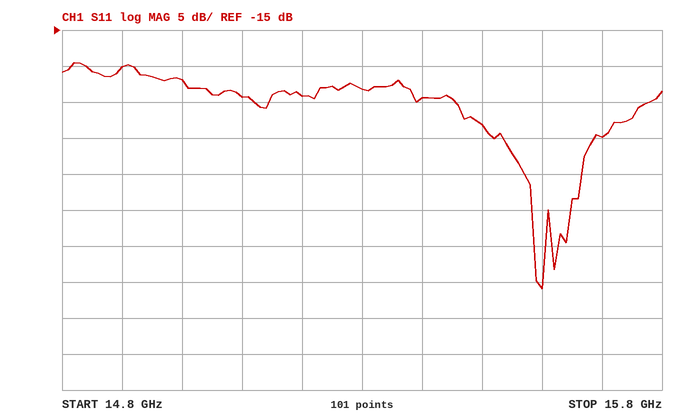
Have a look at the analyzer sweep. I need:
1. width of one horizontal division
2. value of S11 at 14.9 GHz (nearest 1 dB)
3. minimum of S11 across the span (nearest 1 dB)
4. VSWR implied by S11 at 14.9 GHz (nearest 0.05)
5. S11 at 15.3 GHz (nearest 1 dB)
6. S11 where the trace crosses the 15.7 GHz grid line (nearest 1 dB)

100 MHz
-20 dB
-51 dB
1.20
-23 dB
-30 dB
